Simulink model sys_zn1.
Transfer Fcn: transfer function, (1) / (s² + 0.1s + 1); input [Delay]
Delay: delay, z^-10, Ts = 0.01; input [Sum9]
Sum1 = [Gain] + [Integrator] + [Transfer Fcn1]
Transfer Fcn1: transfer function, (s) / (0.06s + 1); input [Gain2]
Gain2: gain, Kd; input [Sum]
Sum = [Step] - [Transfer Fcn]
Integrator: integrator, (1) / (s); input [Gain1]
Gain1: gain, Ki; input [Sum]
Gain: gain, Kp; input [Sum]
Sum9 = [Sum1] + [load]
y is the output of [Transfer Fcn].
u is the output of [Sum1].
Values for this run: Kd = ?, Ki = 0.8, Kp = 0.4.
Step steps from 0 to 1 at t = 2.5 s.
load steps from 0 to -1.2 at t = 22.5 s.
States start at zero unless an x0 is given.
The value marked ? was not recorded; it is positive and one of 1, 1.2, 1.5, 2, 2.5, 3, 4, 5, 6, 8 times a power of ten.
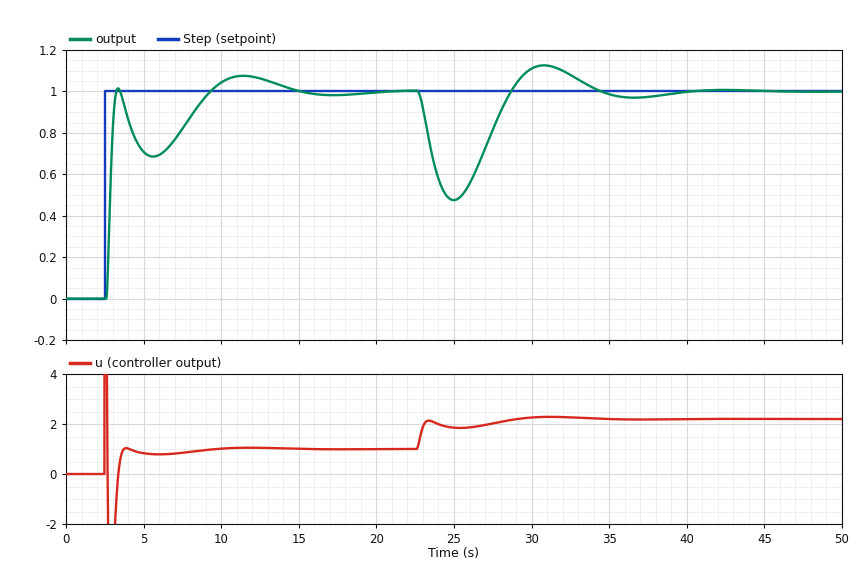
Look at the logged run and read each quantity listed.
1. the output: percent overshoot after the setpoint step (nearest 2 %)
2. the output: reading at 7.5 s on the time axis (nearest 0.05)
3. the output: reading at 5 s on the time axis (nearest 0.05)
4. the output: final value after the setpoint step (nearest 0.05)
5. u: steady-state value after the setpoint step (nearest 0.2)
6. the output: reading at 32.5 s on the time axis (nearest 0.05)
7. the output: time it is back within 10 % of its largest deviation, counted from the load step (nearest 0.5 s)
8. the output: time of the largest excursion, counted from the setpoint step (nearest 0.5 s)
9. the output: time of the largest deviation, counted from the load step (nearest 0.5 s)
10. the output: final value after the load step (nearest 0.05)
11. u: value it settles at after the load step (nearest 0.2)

8 %
0.80
0.70
1.00
1.0
1.10
10.5 s
9.0 s
2.5 s
1.00
2.2
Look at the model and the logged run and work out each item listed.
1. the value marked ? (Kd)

2.5
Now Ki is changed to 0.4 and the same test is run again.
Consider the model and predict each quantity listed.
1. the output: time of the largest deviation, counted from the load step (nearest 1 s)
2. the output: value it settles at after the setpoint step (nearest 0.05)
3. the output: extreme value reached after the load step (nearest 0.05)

3 s
1.00
0.40
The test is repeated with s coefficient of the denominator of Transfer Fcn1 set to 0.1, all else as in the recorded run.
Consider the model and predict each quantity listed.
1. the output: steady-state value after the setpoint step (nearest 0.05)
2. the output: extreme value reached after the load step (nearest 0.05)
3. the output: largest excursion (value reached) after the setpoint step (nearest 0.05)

1.00
0.50
1.05
